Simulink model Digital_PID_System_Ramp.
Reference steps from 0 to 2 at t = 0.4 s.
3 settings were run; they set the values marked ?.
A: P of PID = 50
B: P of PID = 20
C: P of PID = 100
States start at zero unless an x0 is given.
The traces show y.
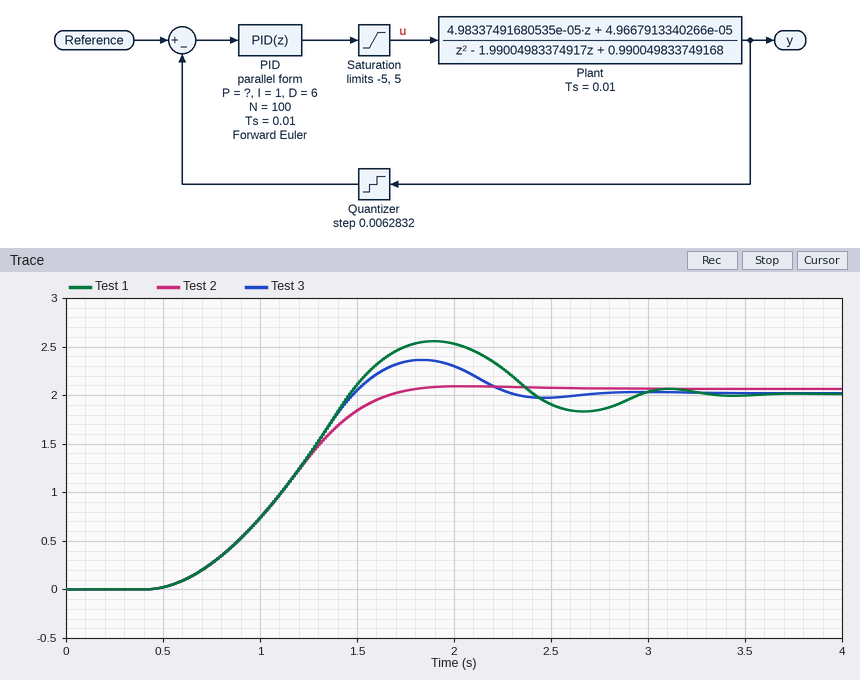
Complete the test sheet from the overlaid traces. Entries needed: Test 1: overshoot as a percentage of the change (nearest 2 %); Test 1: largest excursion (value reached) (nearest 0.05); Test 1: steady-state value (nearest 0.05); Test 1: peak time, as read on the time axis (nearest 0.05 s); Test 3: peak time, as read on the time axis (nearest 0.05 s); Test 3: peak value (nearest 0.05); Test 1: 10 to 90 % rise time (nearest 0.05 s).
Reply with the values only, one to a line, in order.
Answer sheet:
28 %
2.55
2.00
1.90 s
1.85 s
2.35
0.70 s
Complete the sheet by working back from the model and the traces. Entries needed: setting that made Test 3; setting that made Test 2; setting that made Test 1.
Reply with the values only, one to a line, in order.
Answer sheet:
A
B
C
